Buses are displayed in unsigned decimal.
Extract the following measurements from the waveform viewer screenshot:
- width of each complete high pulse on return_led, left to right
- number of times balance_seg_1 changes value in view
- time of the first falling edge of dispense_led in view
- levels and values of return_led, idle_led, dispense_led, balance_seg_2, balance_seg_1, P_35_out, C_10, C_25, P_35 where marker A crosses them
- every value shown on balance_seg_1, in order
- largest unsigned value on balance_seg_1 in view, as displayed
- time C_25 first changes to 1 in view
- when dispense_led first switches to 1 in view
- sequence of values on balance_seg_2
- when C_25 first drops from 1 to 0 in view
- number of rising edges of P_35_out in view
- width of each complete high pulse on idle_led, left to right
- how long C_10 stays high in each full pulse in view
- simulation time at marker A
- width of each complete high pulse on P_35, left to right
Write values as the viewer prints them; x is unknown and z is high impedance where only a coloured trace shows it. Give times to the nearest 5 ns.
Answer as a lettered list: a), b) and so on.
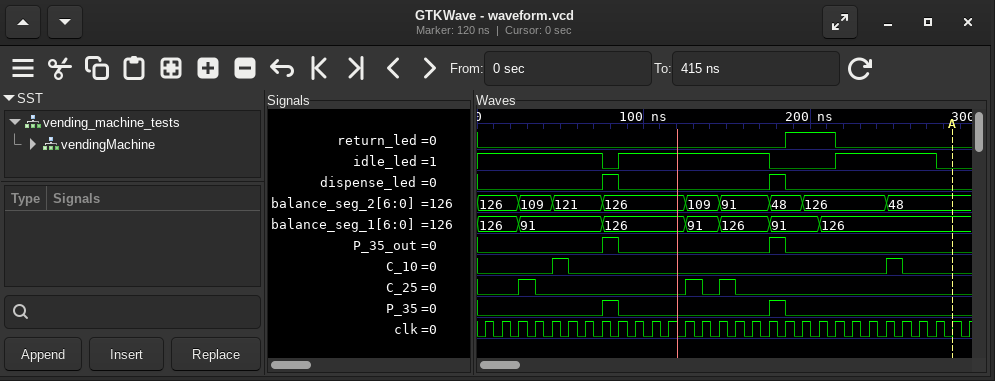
a) 30 ns
b) 6
c) 85 ns
d) return_led=0, idle_led=0, dispense_led=0, balance_seg_2=48, balance_seg_1=126, P_35_out=0, C_10=0, C_25=0, P_35=0
e) 126, 91, 126, 91, 126, 91, 126
f) 126
g) 25 ns
h) 75 ns
i) 126, 109, 121, 126, 109, 91, 48, 126, 48
j) 35 ns
k) 2
l) 90 ns, 60 ns
m) 10 ns, 10 ns
n) 285 ns
o) 10 ns, 10 ns
